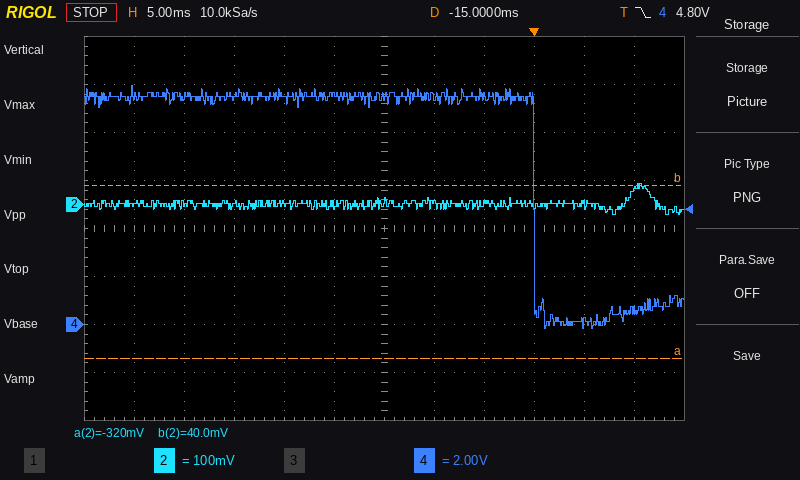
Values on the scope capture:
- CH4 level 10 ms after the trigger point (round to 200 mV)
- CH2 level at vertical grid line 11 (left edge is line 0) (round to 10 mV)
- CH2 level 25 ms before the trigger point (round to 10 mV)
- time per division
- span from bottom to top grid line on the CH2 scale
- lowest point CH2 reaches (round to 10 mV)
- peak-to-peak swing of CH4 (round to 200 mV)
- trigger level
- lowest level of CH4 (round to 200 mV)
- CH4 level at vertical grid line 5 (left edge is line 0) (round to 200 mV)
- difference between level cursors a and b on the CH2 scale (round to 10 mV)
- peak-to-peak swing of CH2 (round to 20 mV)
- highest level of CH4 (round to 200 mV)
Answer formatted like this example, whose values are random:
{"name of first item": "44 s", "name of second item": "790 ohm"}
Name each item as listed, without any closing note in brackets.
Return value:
{"CH4 level 10 ms after the trigger point": "600 mV", "CH2 level at vertical grid line 11 (left edge is line 0)": "30 mV", "CH2 level 25 ms before the trigger point": "0 mV", "time per division": "5 ms", "span from bottom to top grid line on the CH2 scale": "800 mV", "lowest point CH2 reaches": "-20 mV", "peak-to-peak swing of CH4": "10.2 V", "trigger level": "4.80 V", "lowest level of CH4": "-200 mV", "CH4 level at vertical grid line 5 (left edge is line 0)": "9.6 V", "difference between level cursors a and b on the CH2 scale": "360 mV", "peak-to-peak swing of CH2": "60 mV", "highest level of CH4": "10.0 V"}
